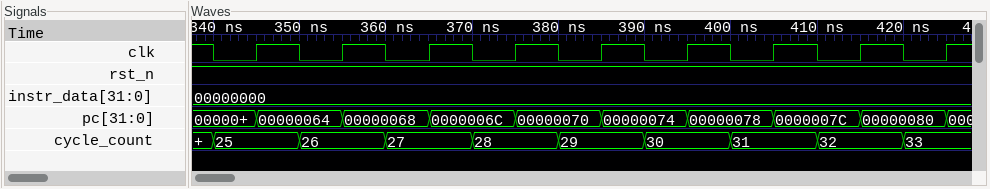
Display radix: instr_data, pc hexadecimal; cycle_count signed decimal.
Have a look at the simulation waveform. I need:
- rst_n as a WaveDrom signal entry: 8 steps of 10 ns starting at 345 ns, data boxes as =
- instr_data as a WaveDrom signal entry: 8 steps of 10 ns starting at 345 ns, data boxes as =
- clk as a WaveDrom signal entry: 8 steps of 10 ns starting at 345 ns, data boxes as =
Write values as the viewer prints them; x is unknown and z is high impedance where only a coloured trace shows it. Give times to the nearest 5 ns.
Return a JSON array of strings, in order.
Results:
["{name: 'rst_n', wave: '1.......'}", "{name: 'instr_data', wave: '=.......', data: '00000000'}", "{name: 'clk', wave: 'p.......'}"]
